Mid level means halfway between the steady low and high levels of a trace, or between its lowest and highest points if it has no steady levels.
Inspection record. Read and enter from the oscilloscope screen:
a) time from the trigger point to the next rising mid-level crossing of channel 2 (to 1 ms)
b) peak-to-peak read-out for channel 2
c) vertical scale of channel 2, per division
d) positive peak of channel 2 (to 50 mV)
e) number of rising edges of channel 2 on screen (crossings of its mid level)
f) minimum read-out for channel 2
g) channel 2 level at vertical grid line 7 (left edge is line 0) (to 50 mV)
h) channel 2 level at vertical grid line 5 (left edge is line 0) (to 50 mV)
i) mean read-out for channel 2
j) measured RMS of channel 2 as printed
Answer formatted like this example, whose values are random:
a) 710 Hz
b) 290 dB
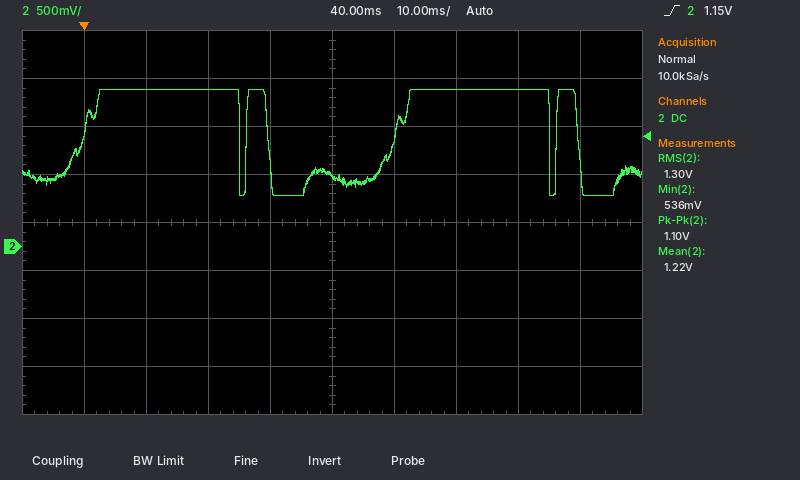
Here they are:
a) 26 ms
b) 1.10 V
c) 500 mV
d) 1.65 V
e) 4
f) 536 mV
g) 1.65 V
h) 750 mV
i) 1.22 V
j) 1.30 V
